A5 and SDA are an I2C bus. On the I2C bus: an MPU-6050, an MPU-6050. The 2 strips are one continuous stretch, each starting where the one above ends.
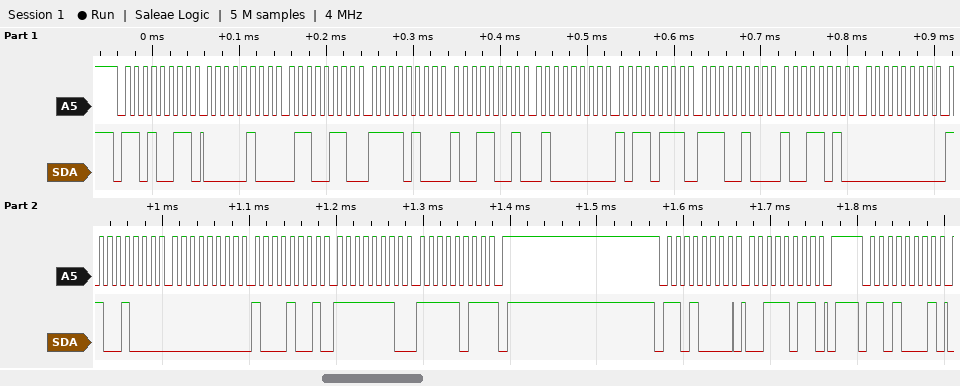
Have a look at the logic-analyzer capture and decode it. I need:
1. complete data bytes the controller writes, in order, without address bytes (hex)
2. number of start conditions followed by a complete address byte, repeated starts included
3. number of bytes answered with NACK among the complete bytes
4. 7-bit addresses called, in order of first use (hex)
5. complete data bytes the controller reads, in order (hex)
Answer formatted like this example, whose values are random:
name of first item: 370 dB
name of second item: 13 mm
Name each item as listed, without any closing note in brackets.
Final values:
complete data bytes the controller writes, in order, without address bytes: 3B
number of start conditions followed by a complete address byte, repeated starts included: 3
number of bytes answered with NACK among the complete bytes: 1
7-bit addresses called, in order of first use: 0x69 0x68
complete data bytes the controller reads, in order: 04 66 F4 99 40 B7 E4 9A 00 C8 00 89 FE FB
